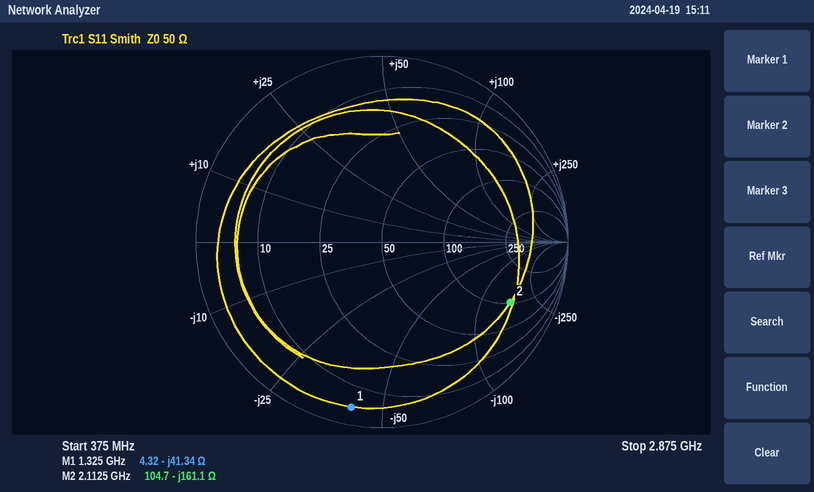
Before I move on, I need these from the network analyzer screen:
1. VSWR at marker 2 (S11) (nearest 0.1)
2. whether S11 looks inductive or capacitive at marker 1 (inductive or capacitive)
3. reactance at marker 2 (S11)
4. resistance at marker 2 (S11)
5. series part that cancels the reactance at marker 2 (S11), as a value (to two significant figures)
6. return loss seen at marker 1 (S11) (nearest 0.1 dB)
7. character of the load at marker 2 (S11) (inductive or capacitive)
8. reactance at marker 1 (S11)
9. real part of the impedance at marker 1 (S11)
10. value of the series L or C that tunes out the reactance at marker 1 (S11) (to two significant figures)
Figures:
7.4
capacitive
-161.1 Ω
104.7 Ω
12 nH
0.9 dB
capacitive
-41.34 Ω
4.32 Ω
5.0 nH
